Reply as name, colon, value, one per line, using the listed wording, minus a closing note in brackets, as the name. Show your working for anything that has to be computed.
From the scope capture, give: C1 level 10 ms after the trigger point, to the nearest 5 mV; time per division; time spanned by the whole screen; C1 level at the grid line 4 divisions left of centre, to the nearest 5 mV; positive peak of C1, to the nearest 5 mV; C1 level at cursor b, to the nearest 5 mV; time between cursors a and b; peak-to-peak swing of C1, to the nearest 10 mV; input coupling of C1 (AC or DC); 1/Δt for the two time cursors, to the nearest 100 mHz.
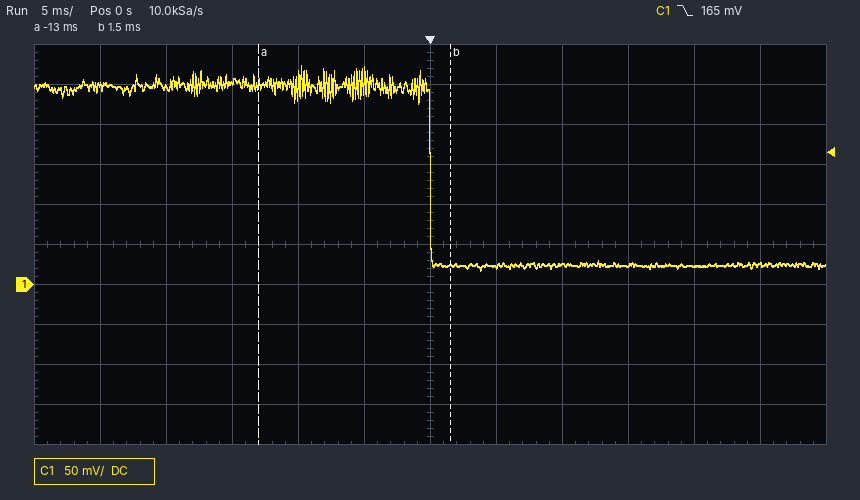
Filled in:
C1 level 10 ms after the trigger point, to the nearest 5 mV: 25 mV
time per division: 5 ms
time spanned by the whole screen: 60 ms
C1 level at the grid line 4 divisions left of centre, to the nearest 5 mV: 245 mV
positive peak of C1, to the nearest 5 mV: 275 mV
C1 level at cursor b, to the nearest 5 mV: 25 mV
time between cursors a and b: 1.5 ms − (-13 ms) = 14.5 ms
peak-to-peak swing of C1, to the nearest 10 mV: 260 mV
input coupling of C1: DC
1/Δt for the two time cursors, to the nearest 100 mHz: 1 / 14.5 ms ≈ 69.0 Hz
